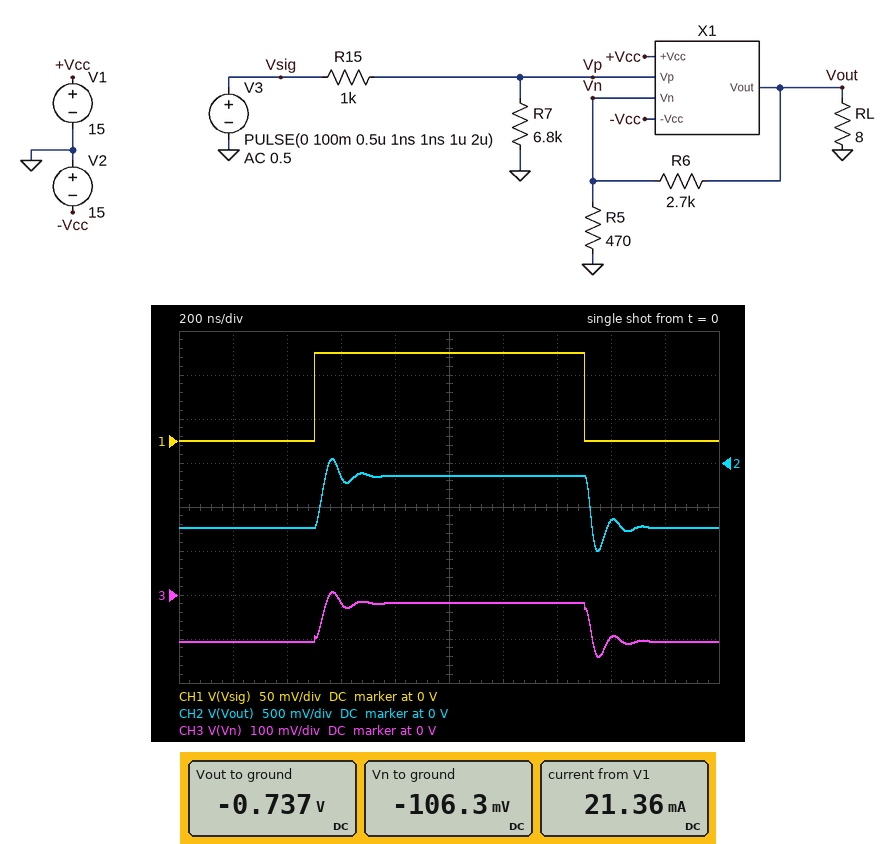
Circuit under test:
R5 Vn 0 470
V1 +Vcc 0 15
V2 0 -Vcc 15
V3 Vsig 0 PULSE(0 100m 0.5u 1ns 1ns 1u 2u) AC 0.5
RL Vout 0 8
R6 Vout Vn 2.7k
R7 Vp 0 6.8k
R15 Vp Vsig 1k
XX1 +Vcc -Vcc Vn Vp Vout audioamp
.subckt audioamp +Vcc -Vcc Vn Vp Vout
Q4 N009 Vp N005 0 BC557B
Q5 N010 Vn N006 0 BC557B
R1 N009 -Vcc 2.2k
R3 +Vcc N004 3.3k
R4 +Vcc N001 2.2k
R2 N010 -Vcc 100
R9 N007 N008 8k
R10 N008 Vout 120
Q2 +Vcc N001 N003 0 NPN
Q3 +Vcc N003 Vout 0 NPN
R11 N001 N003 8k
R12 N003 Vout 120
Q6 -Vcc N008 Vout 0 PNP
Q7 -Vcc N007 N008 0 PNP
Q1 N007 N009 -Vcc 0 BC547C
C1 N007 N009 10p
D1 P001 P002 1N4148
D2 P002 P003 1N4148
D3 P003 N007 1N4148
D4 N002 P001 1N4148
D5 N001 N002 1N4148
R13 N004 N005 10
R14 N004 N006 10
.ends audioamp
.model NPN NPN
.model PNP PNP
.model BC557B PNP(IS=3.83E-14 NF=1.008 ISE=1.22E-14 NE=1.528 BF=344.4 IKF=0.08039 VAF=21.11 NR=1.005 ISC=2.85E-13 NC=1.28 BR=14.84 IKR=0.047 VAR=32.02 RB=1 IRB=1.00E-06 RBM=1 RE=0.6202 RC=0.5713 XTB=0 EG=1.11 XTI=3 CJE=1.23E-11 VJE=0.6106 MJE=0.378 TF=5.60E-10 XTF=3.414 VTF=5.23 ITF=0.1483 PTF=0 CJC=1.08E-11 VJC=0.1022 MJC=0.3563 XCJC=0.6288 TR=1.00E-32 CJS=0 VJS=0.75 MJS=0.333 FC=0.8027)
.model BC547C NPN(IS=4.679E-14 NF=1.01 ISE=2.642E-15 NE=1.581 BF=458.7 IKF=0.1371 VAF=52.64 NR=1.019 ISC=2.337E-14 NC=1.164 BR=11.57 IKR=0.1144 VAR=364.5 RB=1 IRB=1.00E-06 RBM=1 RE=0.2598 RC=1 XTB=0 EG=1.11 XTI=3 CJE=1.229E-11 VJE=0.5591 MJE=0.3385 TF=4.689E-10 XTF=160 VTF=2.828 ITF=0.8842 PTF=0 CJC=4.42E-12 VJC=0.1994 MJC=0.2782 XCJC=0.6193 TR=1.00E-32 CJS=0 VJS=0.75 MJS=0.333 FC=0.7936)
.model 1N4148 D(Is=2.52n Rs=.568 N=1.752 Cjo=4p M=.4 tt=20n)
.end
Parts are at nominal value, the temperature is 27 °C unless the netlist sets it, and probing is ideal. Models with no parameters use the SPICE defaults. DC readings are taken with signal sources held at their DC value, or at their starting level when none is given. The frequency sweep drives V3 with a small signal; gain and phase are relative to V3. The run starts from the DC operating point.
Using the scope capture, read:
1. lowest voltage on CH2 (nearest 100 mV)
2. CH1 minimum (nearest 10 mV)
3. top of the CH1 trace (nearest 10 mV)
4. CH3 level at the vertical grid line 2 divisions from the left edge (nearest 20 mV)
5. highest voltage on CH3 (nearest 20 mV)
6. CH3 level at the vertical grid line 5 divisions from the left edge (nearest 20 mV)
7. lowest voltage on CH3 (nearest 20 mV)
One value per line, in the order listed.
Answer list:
-1.0 V
0 V
100 mV
-100 mV
0 V
-20 mV
-140 mV
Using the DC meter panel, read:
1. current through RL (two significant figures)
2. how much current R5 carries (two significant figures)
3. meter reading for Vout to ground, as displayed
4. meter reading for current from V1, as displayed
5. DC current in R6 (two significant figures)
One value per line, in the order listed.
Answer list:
92 mA
230 µA
-0.737 V
21.36 mA
230 µA
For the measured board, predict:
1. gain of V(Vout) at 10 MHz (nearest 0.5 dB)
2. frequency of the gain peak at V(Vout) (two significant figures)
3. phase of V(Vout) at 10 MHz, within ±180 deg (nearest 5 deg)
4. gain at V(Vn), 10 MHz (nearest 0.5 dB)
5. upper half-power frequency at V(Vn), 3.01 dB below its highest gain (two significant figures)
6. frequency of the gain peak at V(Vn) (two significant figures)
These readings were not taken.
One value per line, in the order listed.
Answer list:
20.0 dB
8.9 MHz
-100 deg
2.5 dB
11 MHz
8.7 MHz
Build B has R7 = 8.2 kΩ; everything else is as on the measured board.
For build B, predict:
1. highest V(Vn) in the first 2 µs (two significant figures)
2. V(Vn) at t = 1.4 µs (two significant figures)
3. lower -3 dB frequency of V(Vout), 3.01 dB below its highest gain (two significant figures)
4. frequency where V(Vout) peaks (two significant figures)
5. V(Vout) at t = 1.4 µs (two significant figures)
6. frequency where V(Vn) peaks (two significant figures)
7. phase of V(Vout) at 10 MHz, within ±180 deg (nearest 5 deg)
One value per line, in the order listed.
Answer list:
9.4 mV
-17 mV
5.3 MHz
8.8 MHz
-130 mV
8.6 MHz
-105 deg
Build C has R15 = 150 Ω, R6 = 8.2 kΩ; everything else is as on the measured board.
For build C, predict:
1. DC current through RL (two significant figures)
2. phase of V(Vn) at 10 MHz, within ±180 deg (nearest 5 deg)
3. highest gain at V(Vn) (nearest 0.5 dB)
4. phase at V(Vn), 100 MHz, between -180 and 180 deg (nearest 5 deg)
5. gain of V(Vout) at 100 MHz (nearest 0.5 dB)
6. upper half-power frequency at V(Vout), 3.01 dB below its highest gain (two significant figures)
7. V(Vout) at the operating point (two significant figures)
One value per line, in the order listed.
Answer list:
250 mA
-95 deg
0 dB
5 deg
-12.0 dB
9.8 MHz
-2.0 V
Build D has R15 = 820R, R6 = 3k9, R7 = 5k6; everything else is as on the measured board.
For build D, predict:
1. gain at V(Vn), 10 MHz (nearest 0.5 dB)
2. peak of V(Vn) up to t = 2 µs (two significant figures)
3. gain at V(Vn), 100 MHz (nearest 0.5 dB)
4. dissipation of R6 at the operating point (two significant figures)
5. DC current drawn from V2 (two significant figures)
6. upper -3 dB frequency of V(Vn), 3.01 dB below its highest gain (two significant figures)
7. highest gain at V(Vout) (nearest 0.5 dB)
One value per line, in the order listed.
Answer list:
-1.0 dB
-1.5 mV
-14.5 dB
210 µW
150 mA
10 MHz
22.0 dB
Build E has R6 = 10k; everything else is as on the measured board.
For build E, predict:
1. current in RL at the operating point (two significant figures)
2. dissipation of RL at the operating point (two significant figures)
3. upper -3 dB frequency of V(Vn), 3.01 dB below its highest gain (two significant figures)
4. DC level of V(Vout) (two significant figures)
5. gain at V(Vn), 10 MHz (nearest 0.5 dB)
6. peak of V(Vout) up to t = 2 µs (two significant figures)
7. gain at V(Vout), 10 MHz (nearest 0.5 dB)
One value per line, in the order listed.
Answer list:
300 mA
740 mW
5.8 MHz
-2.4 V
-16.5 dB
-310 mV
16.0 dB
